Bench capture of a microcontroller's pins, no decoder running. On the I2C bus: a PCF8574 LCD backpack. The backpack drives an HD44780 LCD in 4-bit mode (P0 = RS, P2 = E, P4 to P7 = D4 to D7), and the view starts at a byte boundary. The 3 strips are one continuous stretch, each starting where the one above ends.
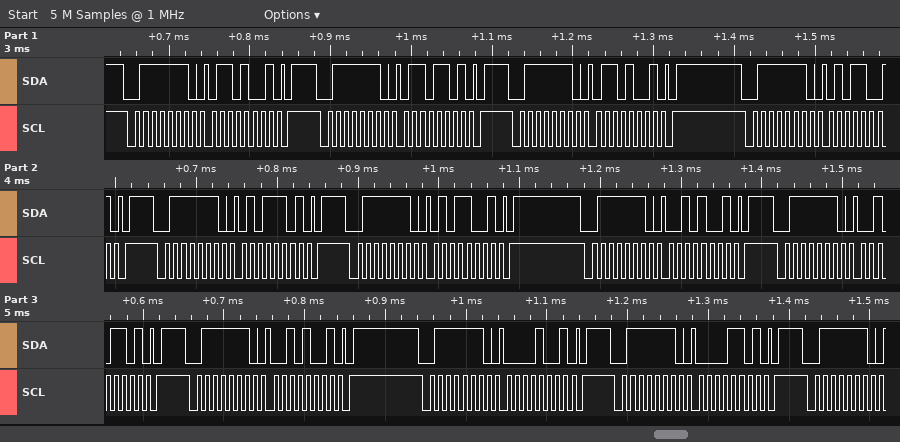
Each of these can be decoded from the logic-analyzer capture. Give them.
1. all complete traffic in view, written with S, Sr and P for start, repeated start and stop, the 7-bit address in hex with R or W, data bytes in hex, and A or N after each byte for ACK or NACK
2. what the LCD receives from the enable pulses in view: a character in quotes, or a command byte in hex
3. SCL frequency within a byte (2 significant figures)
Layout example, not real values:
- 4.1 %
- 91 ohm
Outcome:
- S 3FW A 69 A P S 3FW A 6D A P S 3FW A 69 A P S 3FW A 59 A P S 3FW A 5D A P S 3FW A 59 A P S 3FW A 29 A P S 3FW A 2D A P S 3FW A 29 A P S 3FW A 09 A P S 3FW A 0D A P S 3FW A
- 'e'
- 100 kHz
